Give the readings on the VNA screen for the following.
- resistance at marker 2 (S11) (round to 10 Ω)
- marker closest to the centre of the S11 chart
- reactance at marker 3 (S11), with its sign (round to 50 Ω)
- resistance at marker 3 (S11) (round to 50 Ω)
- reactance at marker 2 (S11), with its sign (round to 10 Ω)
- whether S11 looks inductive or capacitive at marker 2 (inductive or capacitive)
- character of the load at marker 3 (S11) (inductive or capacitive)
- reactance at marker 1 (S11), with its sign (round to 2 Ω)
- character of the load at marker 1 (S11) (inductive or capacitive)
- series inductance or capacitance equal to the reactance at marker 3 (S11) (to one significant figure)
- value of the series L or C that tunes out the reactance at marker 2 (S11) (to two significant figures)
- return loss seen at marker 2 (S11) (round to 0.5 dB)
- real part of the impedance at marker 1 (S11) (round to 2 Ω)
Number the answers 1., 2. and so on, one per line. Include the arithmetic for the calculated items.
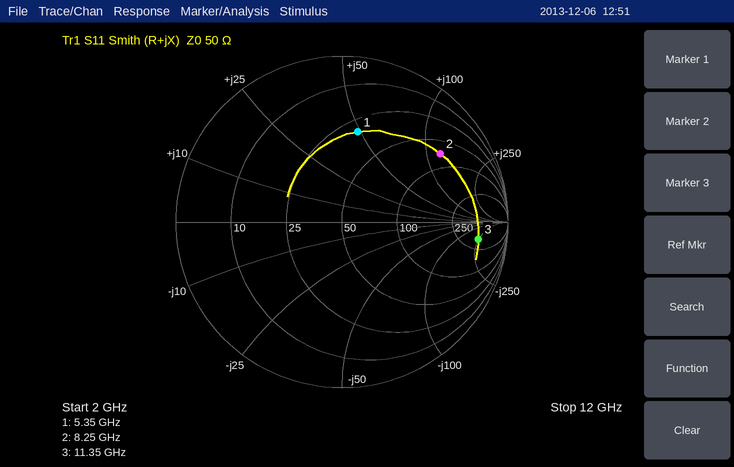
1. 70 Ω
2. marker 1
3. -250 Ω
4. 350 Ω
5. +120 Ω
6. inductive
7. capacitive
8. +48 Ω
9. inductive
10. C = 1/(2π × 11.35 GHz × 250 Ω) ≈ 56.1 fF, so 60 fF to one significant figure
11. C = 1/(2π × 8.25 GHz × 120 Ω) ≈ 161 fF, so 160 fF to two significant figures
12. 3.0 dB
13. 32 Ω
